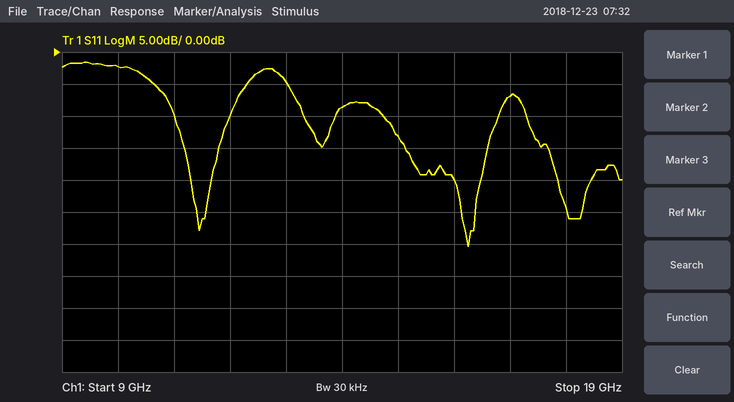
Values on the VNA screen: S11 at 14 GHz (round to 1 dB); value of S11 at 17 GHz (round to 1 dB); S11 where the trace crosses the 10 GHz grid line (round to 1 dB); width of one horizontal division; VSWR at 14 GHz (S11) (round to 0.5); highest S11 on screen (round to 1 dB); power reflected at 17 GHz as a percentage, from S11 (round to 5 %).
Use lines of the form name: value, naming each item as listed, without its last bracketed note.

S11 at 14 GHz: -9 dB
value of S11 at 17 GHz: -7 dB
S11 where the trace crosses the 10 GHz grid line: -2 dB
width of one horizontal division: 1 GHz
VSWR at 14 GHz (S11): 2.0
highest S11 on screen: -2 dB
power reflected at 17 GHz as a percentage, from S11: 20 %
